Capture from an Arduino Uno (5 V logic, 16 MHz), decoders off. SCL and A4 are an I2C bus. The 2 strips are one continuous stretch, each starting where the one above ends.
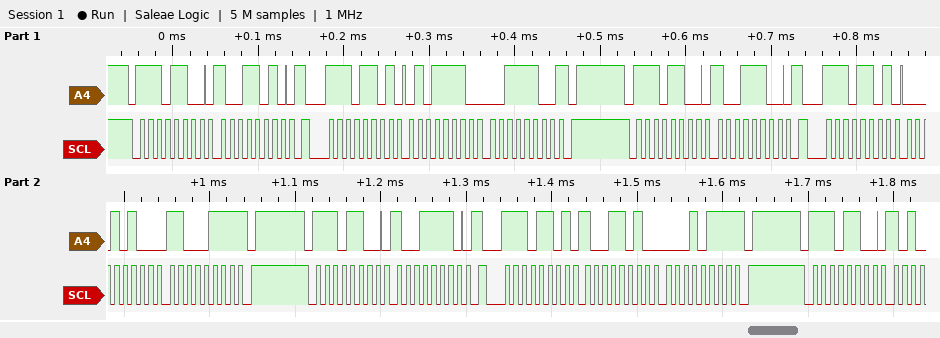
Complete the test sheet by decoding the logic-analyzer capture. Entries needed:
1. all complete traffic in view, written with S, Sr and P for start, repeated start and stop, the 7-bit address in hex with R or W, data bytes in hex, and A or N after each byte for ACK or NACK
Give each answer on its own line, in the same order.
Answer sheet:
S 76W A 9A A Sr 76R A 5E A 3C N P S 76W A 9C A Sr 76R A 14 A C7 N P S 76W A 9E A Sr 76R A 9A A 17 N P S 76W A
